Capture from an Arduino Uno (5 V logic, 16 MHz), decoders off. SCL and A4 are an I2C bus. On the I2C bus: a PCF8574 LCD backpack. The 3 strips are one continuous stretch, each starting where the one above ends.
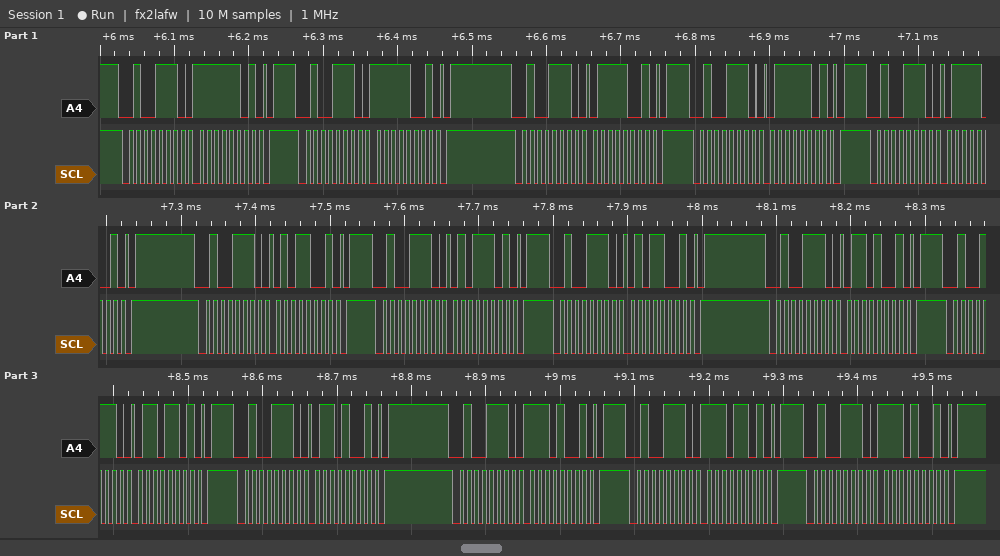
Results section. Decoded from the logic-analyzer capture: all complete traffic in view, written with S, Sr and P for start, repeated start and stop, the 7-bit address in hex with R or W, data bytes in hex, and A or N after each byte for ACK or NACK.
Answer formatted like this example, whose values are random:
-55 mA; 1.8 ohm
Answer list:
S 27W A FD A P S 27W A F9 A P S 27W A 79 A P S 27W A 7D A P S 27W A 79 A P S 27W A 59 A P S 27W A 5D A P S 27W A 59 A P S 27W A 69 A P S 27W A 6D A P S 27W A 69 A P S 27W A E9 A P S 27W A ED A P S 27W A E9 A P
